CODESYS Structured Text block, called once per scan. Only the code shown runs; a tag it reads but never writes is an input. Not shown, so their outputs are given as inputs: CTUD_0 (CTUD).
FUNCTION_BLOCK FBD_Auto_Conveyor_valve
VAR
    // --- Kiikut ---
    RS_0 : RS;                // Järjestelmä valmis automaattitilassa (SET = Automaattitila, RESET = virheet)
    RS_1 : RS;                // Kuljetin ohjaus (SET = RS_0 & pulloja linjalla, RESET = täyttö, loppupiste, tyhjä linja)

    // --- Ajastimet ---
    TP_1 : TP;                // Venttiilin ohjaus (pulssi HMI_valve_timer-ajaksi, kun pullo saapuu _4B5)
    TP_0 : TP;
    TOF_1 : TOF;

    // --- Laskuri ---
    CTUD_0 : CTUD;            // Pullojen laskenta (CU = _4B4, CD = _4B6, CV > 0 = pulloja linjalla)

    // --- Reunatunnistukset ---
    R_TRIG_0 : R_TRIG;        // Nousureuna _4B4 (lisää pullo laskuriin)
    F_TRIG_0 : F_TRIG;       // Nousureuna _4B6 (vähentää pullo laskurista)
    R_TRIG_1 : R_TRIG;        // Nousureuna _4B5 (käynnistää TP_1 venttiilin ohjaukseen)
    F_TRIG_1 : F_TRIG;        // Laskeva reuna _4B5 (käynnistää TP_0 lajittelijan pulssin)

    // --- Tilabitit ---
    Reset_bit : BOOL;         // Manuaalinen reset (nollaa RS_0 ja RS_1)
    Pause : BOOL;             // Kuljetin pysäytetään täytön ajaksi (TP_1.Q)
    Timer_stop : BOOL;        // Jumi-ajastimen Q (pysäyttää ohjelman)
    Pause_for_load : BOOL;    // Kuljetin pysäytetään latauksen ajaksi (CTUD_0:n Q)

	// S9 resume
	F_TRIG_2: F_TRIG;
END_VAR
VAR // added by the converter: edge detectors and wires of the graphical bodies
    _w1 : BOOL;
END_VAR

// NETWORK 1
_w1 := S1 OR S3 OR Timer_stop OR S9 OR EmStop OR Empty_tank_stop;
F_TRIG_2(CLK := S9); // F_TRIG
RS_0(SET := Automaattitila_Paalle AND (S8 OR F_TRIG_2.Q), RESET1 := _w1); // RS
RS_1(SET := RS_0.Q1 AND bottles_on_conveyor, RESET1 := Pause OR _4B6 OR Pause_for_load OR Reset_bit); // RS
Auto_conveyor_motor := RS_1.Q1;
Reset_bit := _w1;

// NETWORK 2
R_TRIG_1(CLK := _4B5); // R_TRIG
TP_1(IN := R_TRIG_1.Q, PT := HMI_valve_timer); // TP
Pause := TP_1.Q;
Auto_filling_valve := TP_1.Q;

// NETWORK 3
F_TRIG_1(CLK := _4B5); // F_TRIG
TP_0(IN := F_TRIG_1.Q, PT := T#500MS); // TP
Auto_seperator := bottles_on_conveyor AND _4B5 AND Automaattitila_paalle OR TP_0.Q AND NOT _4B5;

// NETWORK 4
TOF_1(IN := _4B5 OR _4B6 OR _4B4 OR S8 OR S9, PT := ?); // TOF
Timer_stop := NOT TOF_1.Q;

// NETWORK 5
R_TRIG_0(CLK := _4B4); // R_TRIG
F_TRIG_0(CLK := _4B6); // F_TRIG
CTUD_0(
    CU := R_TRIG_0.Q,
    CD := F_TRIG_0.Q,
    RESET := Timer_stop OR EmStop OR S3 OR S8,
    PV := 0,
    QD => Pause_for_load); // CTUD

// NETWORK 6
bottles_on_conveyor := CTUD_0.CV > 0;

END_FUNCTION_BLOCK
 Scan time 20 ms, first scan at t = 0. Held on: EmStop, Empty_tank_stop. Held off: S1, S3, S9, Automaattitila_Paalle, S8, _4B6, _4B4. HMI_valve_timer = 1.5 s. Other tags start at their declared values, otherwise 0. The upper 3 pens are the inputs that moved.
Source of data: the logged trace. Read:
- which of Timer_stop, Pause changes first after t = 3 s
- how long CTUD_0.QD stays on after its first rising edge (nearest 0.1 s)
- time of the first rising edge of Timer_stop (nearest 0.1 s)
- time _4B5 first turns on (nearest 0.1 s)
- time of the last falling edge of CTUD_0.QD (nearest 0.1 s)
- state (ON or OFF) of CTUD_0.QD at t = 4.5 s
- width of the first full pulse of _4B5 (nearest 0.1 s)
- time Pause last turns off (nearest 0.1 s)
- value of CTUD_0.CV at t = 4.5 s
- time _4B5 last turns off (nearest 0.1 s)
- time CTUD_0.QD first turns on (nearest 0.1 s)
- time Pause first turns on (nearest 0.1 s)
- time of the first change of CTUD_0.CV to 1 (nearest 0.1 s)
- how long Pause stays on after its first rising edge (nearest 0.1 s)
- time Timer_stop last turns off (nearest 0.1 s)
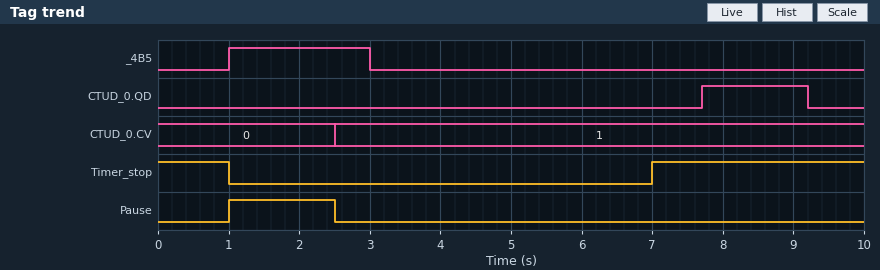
Timer_stop
1.5 s
7.0 s
1.0 s
9.2 s
OFF
2.0 s
2.5 s
1
3.0 s
7.7 s
1.0 s
2.5 s
1.5 s
1.0 s
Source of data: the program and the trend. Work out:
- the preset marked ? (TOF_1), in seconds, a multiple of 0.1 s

4.0 s
